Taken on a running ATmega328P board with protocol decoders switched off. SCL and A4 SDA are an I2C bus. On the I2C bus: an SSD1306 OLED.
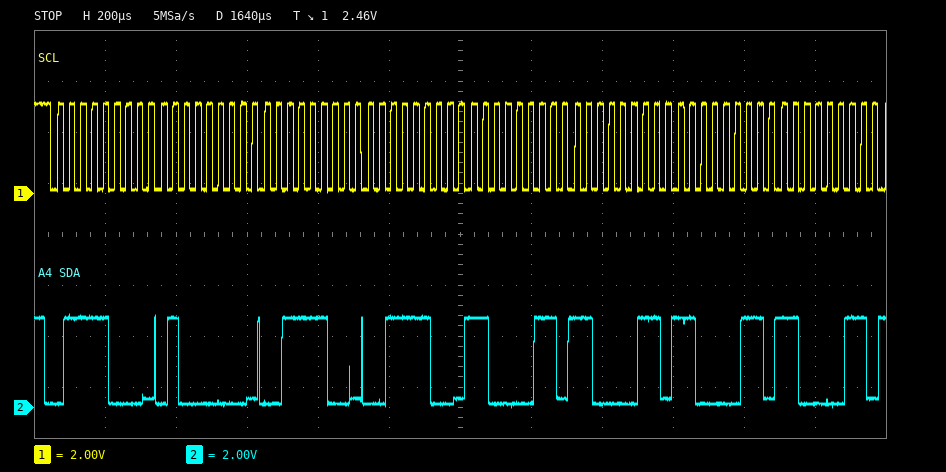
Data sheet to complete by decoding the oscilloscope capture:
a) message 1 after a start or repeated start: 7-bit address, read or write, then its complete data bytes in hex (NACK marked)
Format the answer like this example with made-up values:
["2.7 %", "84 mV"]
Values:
["0x3C write: 40 3C 3C C3 C3 C3 C3"]
